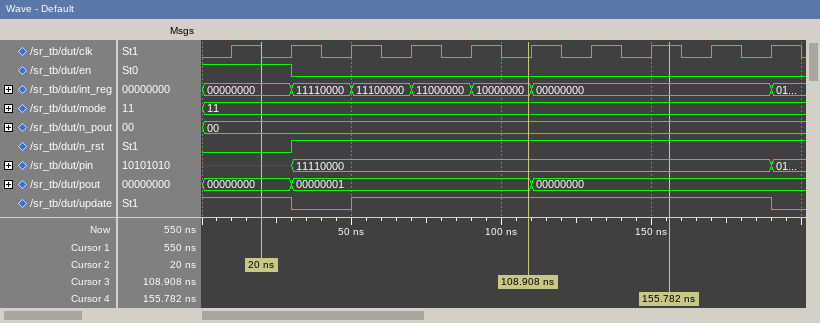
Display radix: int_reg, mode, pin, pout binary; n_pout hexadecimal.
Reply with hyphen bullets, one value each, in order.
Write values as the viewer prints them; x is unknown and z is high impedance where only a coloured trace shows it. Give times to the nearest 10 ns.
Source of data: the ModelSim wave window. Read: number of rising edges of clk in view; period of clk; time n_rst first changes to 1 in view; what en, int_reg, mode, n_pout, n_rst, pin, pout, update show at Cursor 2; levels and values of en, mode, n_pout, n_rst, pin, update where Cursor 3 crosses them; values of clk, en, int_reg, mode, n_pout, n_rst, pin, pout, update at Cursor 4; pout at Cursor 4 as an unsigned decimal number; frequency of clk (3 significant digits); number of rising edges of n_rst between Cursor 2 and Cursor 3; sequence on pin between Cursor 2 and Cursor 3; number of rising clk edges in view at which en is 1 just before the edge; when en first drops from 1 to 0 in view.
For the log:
- 10
- 20 ns
- 30 ns
- en=1, int_reg=00000000, mode=11, n_pout=00, n_rst=0, pin=x, pout=00000000, update=1
- en=0, mode=11, n_pout=00, n_rst=1, pin=11110000, update=1
- clk=1, en=0, int_reg=00000000, mode=11, n_pout=00, n_rst=1, pin=11110000, pout=00000000, update=1
- 0
- 50.0 MHz
- 1
- x, 11110000
- 2
- 30 ns
